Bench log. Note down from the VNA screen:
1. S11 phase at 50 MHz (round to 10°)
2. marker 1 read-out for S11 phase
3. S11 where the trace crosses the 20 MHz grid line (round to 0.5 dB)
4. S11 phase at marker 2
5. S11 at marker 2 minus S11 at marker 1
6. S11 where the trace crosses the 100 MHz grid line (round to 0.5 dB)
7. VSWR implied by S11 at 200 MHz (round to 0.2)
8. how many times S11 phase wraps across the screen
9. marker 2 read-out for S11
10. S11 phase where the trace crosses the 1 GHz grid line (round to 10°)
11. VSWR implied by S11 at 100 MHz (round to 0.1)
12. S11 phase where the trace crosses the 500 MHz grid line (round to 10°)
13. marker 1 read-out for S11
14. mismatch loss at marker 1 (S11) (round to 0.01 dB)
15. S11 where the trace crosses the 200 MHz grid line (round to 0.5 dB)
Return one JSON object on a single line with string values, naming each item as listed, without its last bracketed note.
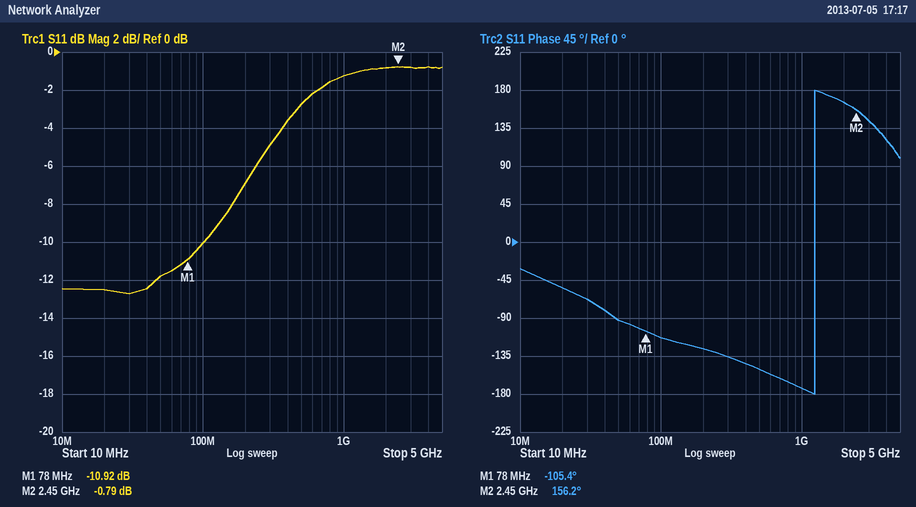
{"S11 phase at 50 MHz": "-90°", "marker 1 read-out for S11 phase": "-105.4°", "S11 where the trace crosses the 20 MHz grid line": "-12.5 dB", "S11 phase at marker 2": "156.2°", "S11 at marker 2 minus S11 at marker 1": "10.13 dB", "S11 where the trace crosses the 100 MHz grid line": "-10.0 dB", "VSWR implied by S11 at 200 MHz": "2.6", "how many times S11 phase wraps across the screen": "1", "marker 2 read-out for S11": "-0.79 dB", "S11 phase where the trace crosses the 1 GHz grid line": "-170°", "VSWR implied by S11 at 100 MHz": "1.9", "S11 phase where the trace crosses the 500 MHz grid line": "-150°", "marker 1 read-out for S11": "-10.92 dB", "mismatch loss at marker 1 (S11)": "0.37 dB", "S11 where the trace crosses the 200 MHz grid line": "-7.0 dB"}
